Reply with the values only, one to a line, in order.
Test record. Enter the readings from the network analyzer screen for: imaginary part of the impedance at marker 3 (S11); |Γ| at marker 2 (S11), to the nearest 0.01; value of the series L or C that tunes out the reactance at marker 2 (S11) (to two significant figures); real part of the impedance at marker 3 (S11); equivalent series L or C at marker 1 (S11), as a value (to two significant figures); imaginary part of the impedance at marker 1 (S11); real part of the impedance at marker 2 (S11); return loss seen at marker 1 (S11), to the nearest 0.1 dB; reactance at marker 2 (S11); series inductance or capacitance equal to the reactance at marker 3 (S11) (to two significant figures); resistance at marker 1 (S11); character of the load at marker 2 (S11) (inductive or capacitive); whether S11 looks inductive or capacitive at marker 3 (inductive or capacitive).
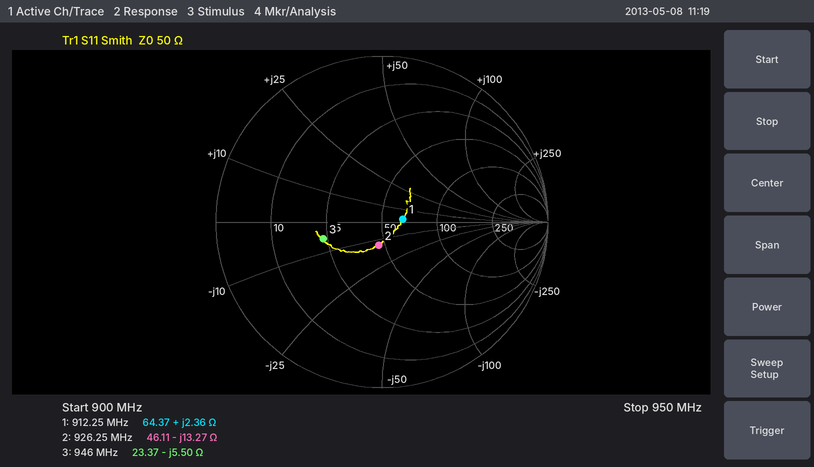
-5.50 Ω
0.14
2.3 nH
23.37 Ω
410 pH
+2.36 Ω
46.11 Ω
17.9 dB
-13.27 Ω
31 pF
64.37 Ω
capacitive
capacitive
